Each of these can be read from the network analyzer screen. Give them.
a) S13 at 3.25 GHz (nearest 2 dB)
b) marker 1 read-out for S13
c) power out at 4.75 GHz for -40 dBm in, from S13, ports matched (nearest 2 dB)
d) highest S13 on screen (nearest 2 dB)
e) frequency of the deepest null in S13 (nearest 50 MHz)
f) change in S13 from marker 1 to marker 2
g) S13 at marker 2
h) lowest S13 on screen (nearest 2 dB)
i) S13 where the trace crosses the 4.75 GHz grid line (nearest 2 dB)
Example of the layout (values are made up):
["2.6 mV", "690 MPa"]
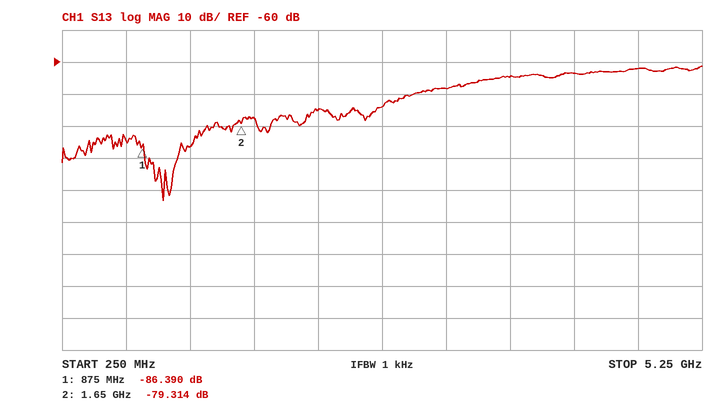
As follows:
["-68 dB", "-86.390 dB", "-102 dBm", "-62 dB", "1.05 GHz", "7.076 dB", "-79.314 dB", "-104 dB", "-62 dB"]
